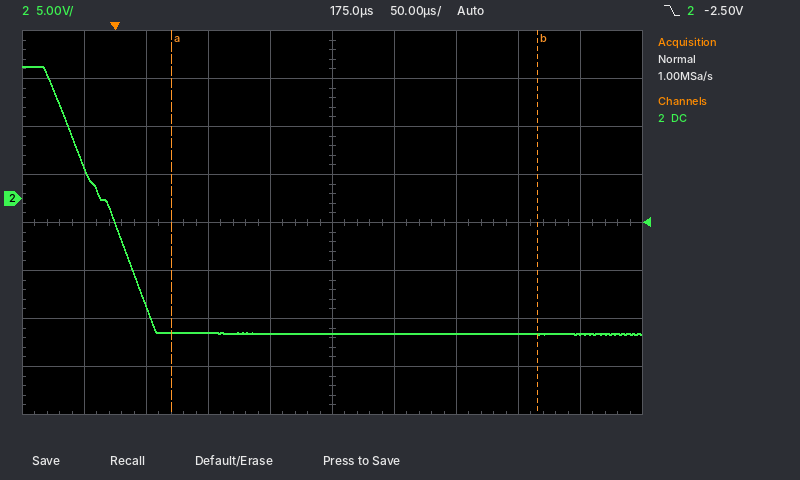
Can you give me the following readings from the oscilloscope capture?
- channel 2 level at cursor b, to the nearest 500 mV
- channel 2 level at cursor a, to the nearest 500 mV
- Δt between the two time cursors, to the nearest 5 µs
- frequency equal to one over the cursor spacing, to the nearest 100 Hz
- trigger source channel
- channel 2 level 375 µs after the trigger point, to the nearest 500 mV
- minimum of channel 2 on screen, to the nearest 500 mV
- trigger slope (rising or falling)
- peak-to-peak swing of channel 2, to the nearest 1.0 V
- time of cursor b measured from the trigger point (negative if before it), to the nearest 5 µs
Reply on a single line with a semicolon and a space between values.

-14.0 V; -14.0 V; 295 µs; 3.4 kHz; channel 2; -14.0 V; -14.0 V; falling; 28.0 V; +340 µs
